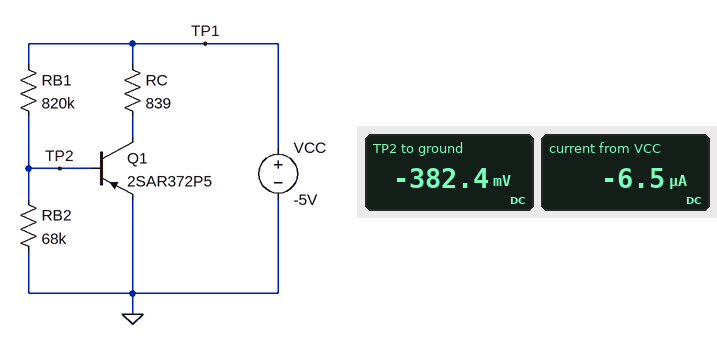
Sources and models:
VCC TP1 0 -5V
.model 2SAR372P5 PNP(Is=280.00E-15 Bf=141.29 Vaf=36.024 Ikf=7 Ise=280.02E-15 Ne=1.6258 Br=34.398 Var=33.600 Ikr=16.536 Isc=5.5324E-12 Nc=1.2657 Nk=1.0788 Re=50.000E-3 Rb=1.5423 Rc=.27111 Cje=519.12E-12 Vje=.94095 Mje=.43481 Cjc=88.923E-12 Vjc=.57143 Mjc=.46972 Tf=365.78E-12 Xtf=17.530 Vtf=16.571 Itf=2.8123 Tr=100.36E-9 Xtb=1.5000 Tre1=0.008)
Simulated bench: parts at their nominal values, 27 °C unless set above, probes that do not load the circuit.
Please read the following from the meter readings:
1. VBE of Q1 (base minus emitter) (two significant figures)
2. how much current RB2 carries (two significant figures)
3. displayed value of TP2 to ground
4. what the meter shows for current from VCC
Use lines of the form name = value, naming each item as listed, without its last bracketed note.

VBE of Q1 (base minus emitter) = -380 mV
how much current RB2 carries = 5.6 µA
displayed value of TP2 to ground = -382.4 mV
what the meter shows for current from VCC = -6.5 µA
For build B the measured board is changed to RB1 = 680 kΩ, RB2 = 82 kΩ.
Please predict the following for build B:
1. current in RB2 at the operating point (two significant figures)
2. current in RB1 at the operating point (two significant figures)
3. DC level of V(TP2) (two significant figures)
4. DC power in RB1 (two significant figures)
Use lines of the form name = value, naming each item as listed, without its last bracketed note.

current in RB2 at the operating point = 6.1 µA
current in RB1 at the operating point = 6.6 µA
DC level of V(TP2) = -500 mV
DC power in RB1 = 30 µW
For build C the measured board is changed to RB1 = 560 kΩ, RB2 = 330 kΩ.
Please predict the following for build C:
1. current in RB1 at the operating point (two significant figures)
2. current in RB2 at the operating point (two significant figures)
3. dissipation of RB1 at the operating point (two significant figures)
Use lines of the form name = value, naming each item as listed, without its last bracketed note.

current in RB1 at the operating point = 7.9 µA
current in RB2 at the operating point = 1.7 µA
dissipation of RB1 at the operating point = 35 µW
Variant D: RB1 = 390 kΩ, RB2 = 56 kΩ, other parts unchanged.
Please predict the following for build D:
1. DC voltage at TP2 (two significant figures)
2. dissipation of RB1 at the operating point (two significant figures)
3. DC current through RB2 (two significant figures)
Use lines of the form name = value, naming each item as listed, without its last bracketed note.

DC voltage at TP2 = -530 mV
dissipation of RB1 at the operating point = 51 µW
DC current through RB2 = 9.5 µA
